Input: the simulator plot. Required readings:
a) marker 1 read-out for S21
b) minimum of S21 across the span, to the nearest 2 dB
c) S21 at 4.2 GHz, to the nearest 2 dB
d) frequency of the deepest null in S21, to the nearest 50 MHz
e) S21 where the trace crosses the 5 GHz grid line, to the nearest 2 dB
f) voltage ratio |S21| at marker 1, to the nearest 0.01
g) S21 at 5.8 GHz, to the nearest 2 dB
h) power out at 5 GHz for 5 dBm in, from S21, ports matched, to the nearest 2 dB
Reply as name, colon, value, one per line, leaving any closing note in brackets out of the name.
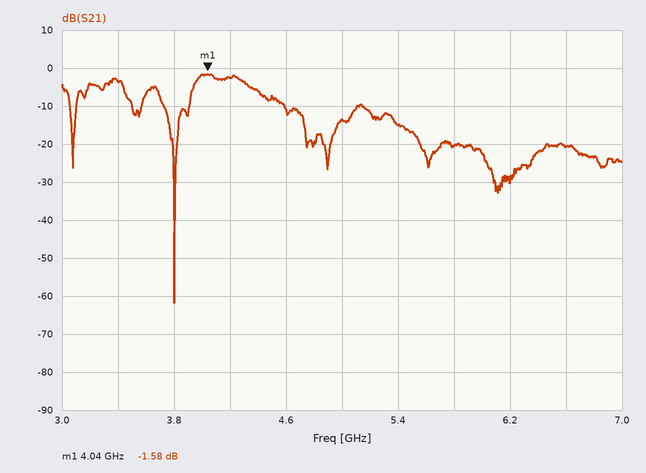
marker 1 read-out for S21: -1.58 dB
minimum of S21 across the span, to the nearest 2 dB: -62 dB
S21 at 4.2 GHz, to the nearest 2 dB: -2 dB
frequency of the deepest null in S21, to the nearest 50 MHz: 3.80 GHz
S21 where the trace crosses the 5 GHz grid line, to the nearest 2 dB: -14 dB
voltage ratio |S21| at marker 1, to the nearest 0.01: 0.83
S21 at 5.8 GHz, to the nearest 2 dB: -20 dB
power out at 5 GHz for 5 dBm in, from S21, ports matched, to the nearest 2 dB: -8 dBm
